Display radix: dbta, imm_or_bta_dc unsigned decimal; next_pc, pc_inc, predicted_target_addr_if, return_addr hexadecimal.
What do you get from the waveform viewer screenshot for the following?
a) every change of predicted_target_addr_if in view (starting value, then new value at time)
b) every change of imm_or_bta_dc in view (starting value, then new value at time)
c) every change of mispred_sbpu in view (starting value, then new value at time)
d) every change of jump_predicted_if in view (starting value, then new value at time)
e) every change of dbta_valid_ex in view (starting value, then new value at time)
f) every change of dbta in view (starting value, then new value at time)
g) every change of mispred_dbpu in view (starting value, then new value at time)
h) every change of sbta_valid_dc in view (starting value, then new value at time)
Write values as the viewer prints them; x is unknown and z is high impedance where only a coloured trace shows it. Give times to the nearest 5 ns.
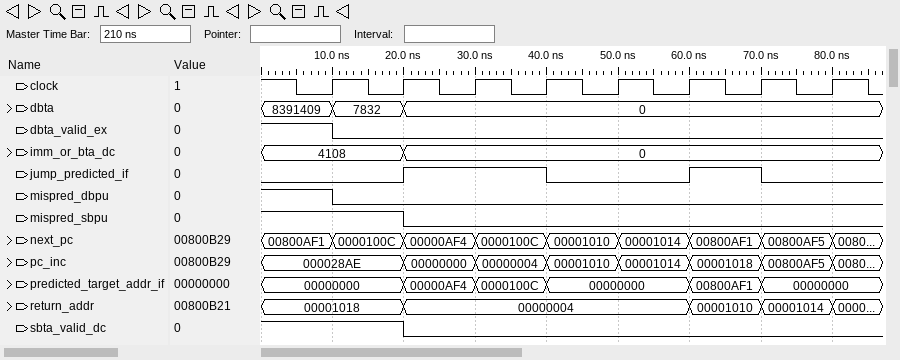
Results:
00000000, 00000AF4 at 20 ns, 0000100C at 30 ns, 00000000 at 40 ns, 00800AF1 at 60 ns, 00000000 at 70 ns
4108, 0 at 20 ns
1, 0 at 20 ns
0, 1 at 20 ns, 0 at 40 ns, 1 at 60 ns, 0 at 70 ns
1, 0 at 10 ns
8391409, 7832 at 10 ns, 0 at 20 ns
1, 0 at 10 ns
1, 0 at 20 ns
